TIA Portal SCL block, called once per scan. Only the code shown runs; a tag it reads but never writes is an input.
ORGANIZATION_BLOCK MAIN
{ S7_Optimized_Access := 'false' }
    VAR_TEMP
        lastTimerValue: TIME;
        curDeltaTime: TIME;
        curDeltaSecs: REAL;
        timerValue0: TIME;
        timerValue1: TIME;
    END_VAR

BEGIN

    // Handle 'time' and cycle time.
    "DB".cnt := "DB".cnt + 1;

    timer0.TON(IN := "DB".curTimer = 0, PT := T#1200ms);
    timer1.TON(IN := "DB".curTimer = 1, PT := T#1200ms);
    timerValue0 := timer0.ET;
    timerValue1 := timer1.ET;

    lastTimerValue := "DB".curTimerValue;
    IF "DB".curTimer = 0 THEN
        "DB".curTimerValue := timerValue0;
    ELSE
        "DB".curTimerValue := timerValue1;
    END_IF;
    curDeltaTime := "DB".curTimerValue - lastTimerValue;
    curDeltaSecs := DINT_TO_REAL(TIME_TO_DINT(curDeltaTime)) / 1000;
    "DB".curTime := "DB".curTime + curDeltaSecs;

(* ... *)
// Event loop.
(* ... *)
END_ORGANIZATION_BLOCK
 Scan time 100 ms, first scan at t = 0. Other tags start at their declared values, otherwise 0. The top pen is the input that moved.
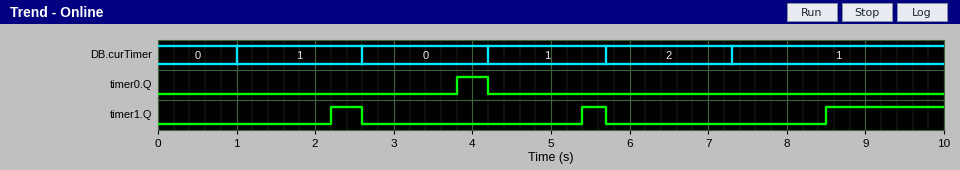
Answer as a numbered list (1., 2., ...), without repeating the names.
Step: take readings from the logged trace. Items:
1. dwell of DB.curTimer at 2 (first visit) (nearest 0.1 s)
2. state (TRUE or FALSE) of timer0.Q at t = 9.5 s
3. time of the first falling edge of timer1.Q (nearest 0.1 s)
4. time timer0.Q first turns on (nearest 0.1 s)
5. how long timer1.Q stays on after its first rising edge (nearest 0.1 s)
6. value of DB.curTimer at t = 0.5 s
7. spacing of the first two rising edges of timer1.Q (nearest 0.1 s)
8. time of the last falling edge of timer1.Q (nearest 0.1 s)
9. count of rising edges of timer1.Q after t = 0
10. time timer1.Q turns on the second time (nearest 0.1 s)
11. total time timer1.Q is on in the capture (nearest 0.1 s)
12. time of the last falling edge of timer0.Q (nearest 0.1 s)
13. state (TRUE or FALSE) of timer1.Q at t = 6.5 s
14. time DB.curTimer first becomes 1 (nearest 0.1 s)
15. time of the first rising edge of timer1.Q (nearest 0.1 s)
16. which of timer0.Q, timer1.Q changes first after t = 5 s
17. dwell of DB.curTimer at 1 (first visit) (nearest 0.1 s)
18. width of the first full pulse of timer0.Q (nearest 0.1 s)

1. 1.6 s
2. FALSE
3. 2.6 s
4. 3.8 s
5. 0.4 s
6. 0
7. 3.2 s
8. 5.7 s
9. 3
10. 5.4 s
11. 2.2 s
12. 4.2 s
13. FALSE
14. 1.0 s
15. 2.2 s
16. timer1.Q
17. 1.6 s
18. 0.4 s
